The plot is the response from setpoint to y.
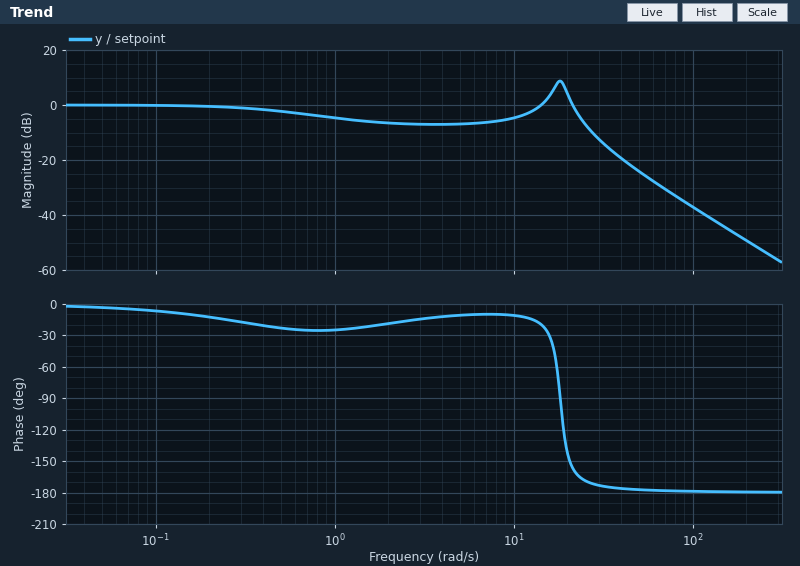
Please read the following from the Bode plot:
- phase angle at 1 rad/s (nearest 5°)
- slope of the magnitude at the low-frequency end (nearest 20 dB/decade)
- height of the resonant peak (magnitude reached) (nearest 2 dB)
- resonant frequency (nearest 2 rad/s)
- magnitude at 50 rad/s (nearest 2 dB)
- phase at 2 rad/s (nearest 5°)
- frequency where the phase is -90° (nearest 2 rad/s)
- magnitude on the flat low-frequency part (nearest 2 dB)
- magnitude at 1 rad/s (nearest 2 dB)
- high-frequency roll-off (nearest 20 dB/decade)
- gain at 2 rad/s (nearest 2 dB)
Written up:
-25°
0 dB/decade
8 dB
18 rad/s
-24 dB
-20°
18 rad/s
0 dB
-4 dB
-40 dB/decade
-6 dB
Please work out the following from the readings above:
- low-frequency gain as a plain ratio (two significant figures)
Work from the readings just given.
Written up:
1.0
